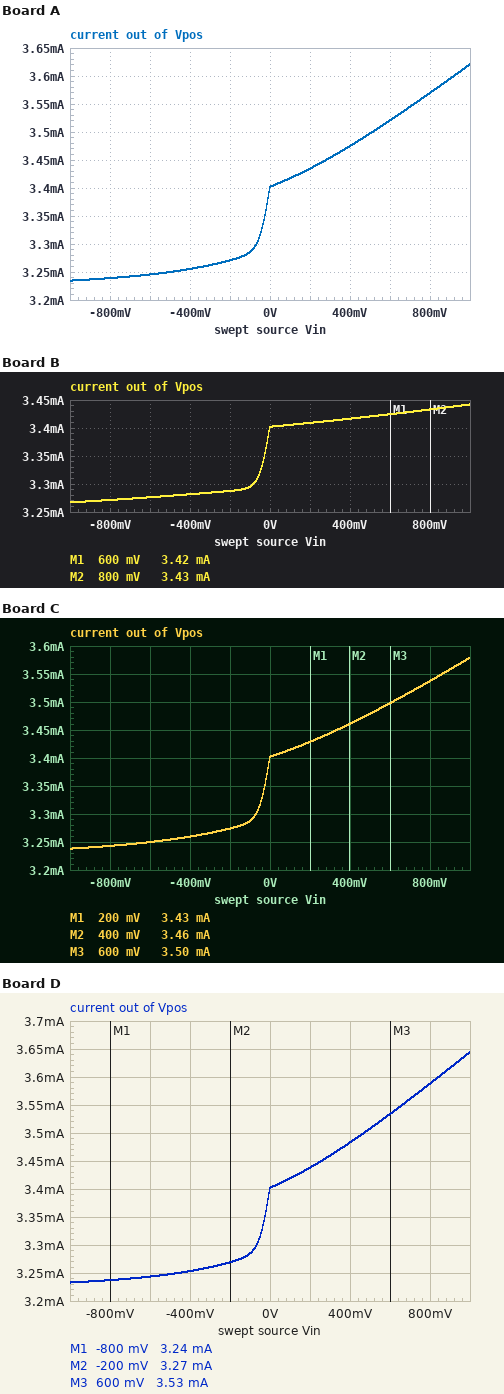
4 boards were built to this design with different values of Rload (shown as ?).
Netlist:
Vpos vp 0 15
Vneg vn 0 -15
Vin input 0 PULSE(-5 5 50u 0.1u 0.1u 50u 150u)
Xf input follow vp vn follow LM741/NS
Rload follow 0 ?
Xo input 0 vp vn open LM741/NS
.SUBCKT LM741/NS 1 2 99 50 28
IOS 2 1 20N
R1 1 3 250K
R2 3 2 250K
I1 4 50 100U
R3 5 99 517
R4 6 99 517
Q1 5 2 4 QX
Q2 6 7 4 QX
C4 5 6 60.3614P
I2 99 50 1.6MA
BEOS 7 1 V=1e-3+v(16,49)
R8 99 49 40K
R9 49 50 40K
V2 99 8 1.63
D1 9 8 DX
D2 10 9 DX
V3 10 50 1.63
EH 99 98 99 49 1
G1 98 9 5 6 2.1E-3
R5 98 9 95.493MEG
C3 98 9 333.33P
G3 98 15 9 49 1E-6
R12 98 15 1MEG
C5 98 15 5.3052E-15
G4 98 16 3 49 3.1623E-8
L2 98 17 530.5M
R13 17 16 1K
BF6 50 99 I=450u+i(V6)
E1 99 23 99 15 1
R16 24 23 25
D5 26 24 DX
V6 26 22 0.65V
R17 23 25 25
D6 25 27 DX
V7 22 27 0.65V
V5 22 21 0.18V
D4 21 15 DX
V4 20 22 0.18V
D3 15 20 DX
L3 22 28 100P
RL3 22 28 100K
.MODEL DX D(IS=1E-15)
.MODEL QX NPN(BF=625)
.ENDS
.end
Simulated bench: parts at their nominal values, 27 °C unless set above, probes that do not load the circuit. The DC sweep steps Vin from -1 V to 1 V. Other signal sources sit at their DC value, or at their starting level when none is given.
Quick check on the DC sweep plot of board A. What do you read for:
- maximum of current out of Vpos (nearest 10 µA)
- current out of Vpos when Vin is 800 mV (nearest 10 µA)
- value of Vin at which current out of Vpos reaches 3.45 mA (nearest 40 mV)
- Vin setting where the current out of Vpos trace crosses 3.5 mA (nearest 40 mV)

3.62 mA
3.57 mA
280 mV
520 mV
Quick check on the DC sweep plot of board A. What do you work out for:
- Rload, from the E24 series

3.6 kΩ
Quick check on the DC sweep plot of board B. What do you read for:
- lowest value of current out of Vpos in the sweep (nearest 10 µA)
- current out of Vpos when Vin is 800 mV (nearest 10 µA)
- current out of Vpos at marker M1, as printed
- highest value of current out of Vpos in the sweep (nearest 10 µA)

3.27 mA
3.43 mA
3.42 mA
3.44 mA
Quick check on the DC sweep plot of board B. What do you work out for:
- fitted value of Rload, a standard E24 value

15 kΩ
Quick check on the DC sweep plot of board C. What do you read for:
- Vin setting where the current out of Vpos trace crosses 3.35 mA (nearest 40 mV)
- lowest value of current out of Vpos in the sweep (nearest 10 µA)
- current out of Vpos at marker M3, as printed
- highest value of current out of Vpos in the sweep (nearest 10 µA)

-40 mV
3.24 mA
3.50 mA
3.58 mA
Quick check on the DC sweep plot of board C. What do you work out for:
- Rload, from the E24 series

4.3 kΩ
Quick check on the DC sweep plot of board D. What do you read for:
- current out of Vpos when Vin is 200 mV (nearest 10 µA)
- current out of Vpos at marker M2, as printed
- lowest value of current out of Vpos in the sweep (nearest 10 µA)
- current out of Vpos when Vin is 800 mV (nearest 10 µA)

3.44 mA
3.27 mA
3.23 mA
3.59 mA
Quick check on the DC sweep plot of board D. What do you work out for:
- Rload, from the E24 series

3.3 kΩ
